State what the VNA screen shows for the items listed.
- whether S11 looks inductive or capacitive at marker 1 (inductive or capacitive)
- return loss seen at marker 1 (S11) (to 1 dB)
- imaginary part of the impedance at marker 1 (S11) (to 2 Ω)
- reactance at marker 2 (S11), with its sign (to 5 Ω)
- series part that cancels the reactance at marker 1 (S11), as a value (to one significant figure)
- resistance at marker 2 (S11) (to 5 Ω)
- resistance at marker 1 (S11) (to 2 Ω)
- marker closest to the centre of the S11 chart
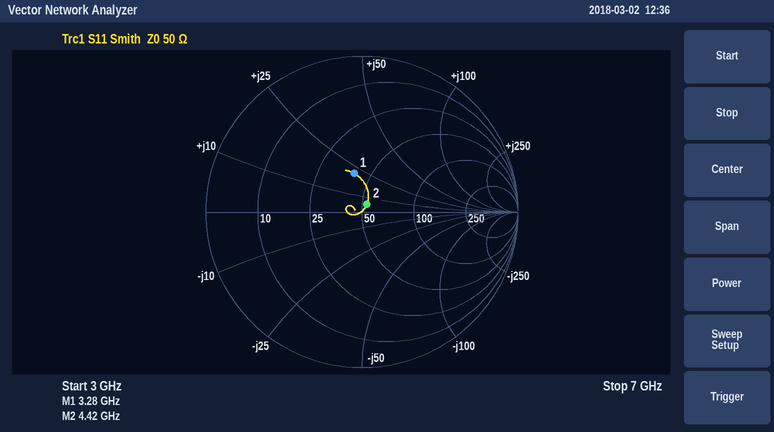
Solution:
inductive
12 dB
+22 Ω
+5 Ω
2 pF
55 Ω
40 Ω
marker 2
